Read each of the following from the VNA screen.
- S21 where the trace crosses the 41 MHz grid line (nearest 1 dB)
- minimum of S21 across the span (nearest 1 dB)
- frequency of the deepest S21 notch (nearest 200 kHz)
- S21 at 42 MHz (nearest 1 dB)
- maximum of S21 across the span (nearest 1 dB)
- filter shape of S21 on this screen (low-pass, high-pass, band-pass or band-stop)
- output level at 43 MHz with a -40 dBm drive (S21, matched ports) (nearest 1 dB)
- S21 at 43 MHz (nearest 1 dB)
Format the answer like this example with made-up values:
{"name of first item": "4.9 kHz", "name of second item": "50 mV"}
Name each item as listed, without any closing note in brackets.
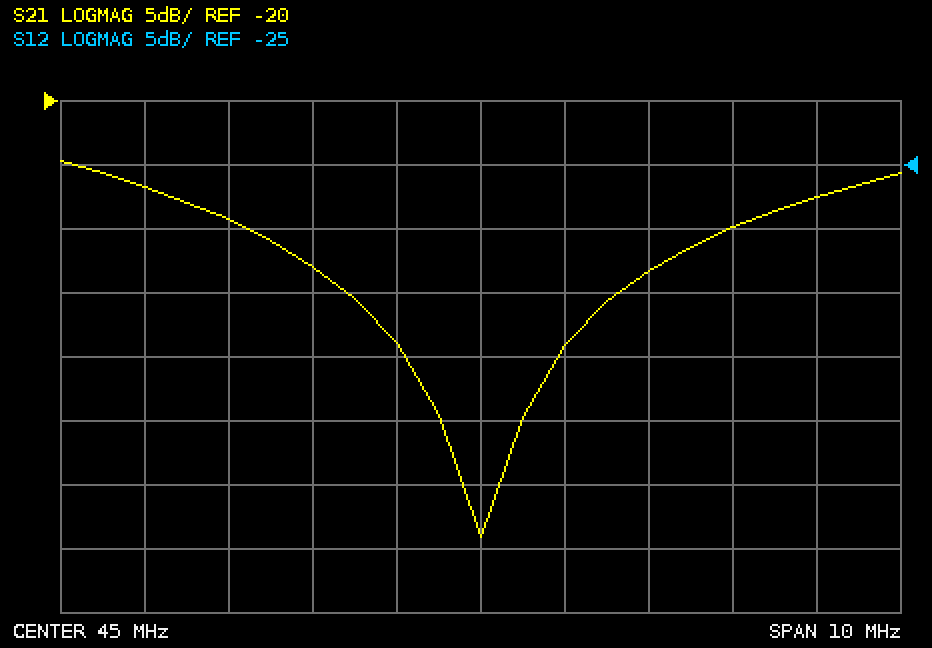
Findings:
{"S21 where the trace crosses the 41 MHz grid line": "-27 dB", "minimum of S21 across the span": "-54 dB", "frequency of the deepest S21 notch": "45.0 MHz", "S21 at 42 MHz": "-29 dB", "maximum of S21 across the span": "-25 dB", "filter shape of S21 on this screen": "band-stop", "output level at 43 MHz with a -40 dBm drive (S21, matched ports)": "-73 dBm", "S21 at 43 MHz": "-33 dB"}
